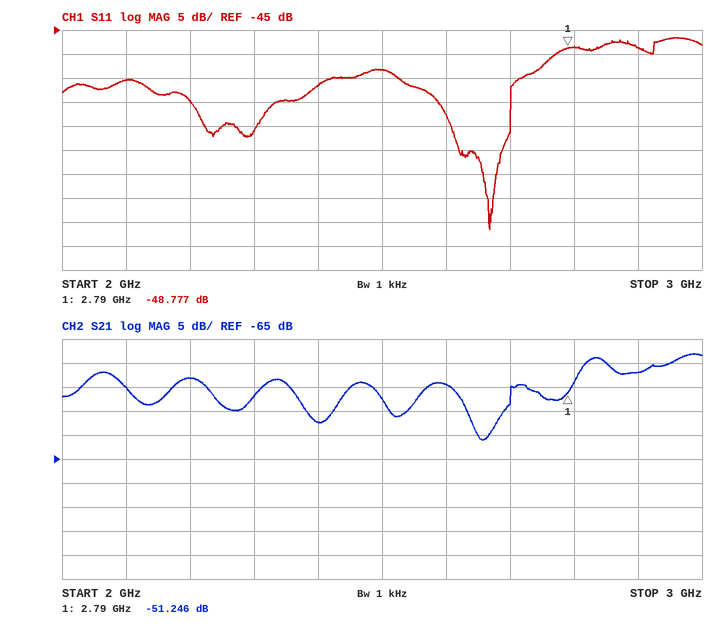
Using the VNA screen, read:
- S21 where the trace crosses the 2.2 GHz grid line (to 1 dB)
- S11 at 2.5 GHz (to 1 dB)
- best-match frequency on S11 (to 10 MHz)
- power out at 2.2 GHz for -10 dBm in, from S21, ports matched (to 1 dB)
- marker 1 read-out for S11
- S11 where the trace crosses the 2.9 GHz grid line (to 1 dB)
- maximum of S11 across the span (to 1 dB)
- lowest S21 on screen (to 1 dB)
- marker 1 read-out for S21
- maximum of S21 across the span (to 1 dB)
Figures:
-48 dB
-53 dB
2.67 GHz
-58 dBm
-48.777 dB
-49 dB
-47 dB
-61 dB
-51.246 dB
-43 dB
